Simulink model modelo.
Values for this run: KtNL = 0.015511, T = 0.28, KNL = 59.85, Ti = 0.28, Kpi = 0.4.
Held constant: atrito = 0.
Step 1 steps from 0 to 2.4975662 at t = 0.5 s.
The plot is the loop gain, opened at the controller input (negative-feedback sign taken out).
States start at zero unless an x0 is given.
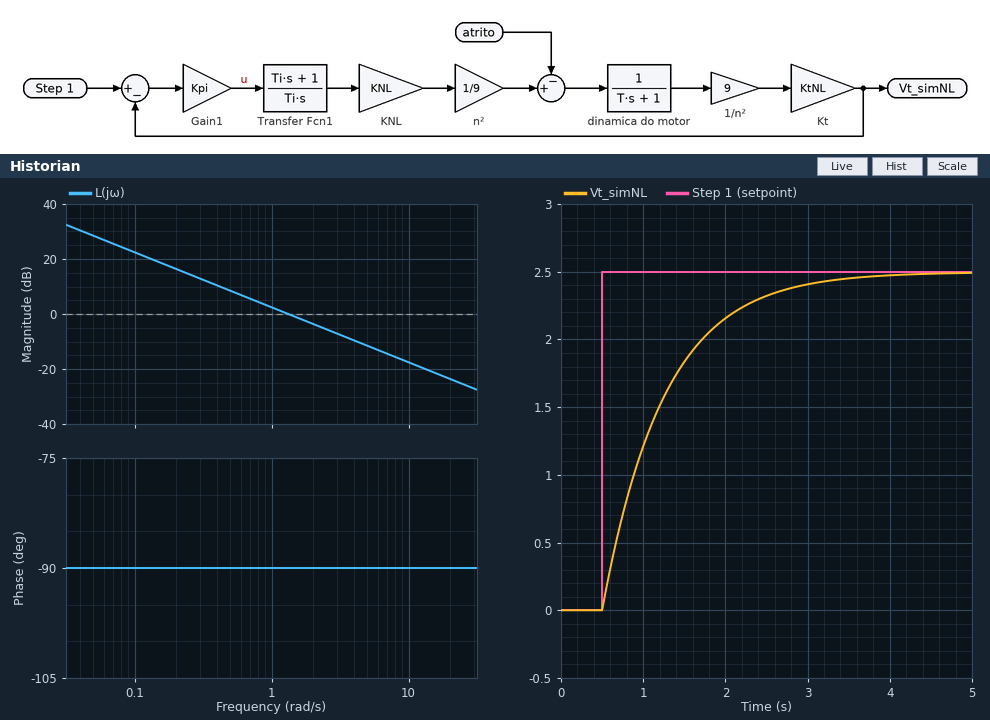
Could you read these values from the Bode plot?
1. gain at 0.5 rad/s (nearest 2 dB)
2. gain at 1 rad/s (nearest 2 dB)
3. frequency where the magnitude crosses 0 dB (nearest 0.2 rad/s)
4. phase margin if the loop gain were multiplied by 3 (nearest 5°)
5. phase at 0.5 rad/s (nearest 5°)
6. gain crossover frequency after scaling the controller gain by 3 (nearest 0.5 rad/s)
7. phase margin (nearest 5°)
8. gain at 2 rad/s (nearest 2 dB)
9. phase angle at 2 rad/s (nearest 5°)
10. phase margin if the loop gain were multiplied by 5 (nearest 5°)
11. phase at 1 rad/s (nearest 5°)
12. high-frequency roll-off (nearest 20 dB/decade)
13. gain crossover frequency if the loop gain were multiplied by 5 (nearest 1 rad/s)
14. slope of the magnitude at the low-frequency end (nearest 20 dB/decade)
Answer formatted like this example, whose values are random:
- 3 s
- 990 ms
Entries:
- 8 dB
- 2 dB
- 1.4 rad/s
- 90°
- -90°
- 4.0 rad/s
- 90°
- -4 dB
- -90°
- 90°
- -90°
- -20 dB/decade
- 7 rad/s
- -20 dB/decade
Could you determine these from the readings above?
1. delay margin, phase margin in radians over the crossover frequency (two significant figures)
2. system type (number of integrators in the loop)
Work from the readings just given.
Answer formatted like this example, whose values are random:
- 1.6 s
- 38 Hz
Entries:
- 1.1 s
- 1
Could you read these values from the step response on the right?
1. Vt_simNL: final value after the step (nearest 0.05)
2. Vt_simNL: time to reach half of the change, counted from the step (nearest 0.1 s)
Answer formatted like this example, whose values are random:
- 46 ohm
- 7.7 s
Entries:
- 2.50
- 0.5 s
